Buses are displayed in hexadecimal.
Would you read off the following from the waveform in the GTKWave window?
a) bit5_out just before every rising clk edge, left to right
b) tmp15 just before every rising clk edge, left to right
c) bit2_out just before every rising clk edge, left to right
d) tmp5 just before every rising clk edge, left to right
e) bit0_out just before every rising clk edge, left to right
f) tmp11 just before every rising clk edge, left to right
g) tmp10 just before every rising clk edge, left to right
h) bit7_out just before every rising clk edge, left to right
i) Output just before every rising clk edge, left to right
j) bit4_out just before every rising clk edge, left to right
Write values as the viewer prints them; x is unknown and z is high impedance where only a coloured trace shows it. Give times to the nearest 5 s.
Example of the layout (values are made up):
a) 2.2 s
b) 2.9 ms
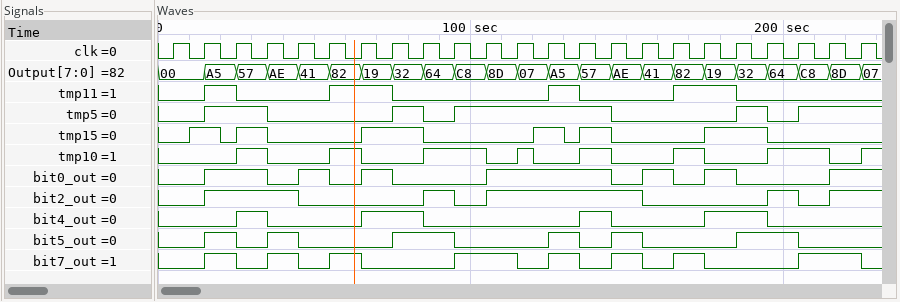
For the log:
a) 0 0 1 0 1 0 0 0 1 1 0 0 0 1 0 1 0 0 0 1 1 0 0
b) 0 1 0 1 0 0 0 1 1 0 0 0 1 0 1 0 0 0 1 1 0 0 0
c) 0 0 1 1 1 0 0 0 0 1 0 1 1 1 1 1 0 0 0 0 1 0 1
d) 0 0 1 1 0 0 0 0 1 0 1 1 1 1 1 0 0 0 0 1 0 1 1
e) 0 0 1 1 0 1 0 1 0 0 0 1 1 1 1 0 1 0 1 0 0 0 1
f) 0 0 1 0 0 0 1 1 0 0 0 0 0 1 0 0 0 1 1 0 0 0 0
g) 0 0 0 1 0 0 1 0 0 1 1 0 0 0 1 0 0 1 0 0 1 1 0
h) 0 0 1 0 1 0 1 0 0 0 1 1 0 1 0 1 0 1 0 0 0 1 1
i) 00, 00, A5, 57, AE, 41, 82, 19, 32, 64, C8, 8D, 07, A5, 57, AE, 41, 82, 19, 32, 64, C8, 8D
j) 0 0 0 1 0 0 0 1 1 0 0 0 0 0 1 0 0 0 1 1 0 0 0
